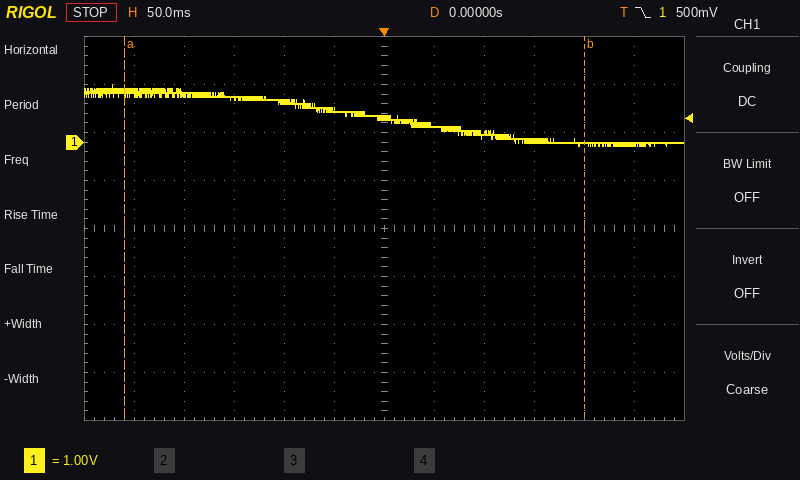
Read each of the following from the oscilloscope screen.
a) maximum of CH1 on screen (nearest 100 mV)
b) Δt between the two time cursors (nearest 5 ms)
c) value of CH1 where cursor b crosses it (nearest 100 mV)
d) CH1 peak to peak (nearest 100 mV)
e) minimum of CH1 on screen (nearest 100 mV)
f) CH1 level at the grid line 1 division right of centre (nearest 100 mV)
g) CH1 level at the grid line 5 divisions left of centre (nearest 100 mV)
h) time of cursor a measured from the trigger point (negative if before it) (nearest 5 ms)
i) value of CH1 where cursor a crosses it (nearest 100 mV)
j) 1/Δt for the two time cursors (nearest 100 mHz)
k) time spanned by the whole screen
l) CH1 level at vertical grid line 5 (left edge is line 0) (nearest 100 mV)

1.2 V
460 ms
0.0 V
1.3 V
-100 mV
300 mV
1.0 V
-260 ms
1.0 V
2.2 Hz
600 ms
700 mV
